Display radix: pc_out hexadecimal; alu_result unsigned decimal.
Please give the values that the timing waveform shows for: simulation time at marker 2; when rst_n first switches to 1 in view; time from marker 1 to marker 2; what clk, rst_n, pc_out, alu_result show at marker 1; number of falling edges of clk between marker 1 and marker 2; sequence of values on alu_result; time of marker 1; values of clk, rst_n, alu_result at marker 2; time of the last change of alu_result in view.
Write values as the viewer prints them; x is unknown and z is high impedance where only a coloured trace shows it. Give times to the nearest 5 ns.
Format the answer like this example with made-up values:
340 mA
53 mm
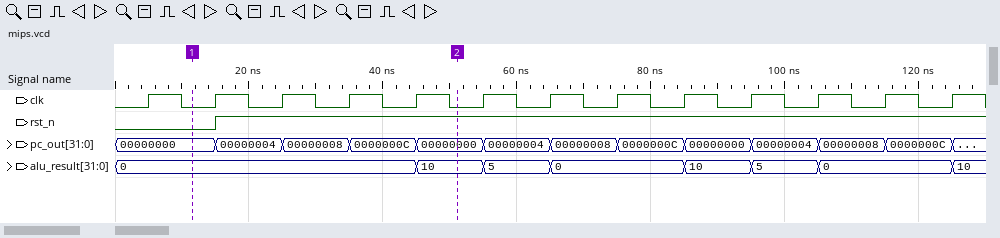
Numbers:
50 ns
15 ns
40 ns
clk=0, rst_n=0, pc_out=00000000, alu_result=0
4
0, 10, 5, 0, 10, 5, 0, 10
10 ns
clk=0, rst_n=1, alu_result=10
125 ns
